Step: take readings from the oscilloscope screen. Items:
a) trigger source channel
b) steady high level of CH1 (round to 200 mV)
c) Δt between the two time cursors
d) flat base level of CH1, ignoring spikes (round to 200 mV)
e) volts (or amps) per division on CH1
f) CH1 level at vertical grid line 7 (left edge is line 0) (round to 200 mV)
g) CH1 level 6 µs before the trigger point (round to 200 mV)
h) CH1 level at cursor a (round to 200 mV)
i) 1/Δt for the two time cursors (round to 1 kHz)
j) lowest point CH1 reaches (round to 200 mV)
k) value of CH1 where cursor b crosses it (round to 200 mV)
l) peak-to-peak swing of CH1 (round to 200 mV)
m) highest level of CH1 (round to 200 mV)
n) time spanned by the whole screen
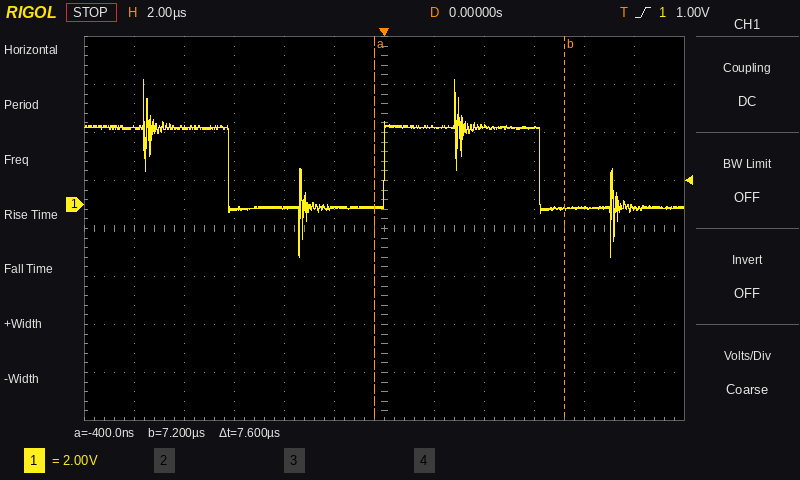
CH1
3.2 V
7.6 µs
-200 mV
2 V
3.2 V
-200 mV
-200 mV
132 kHz
-2.2 V
-200 mV
7.4 V
5.2 V
24 µs
